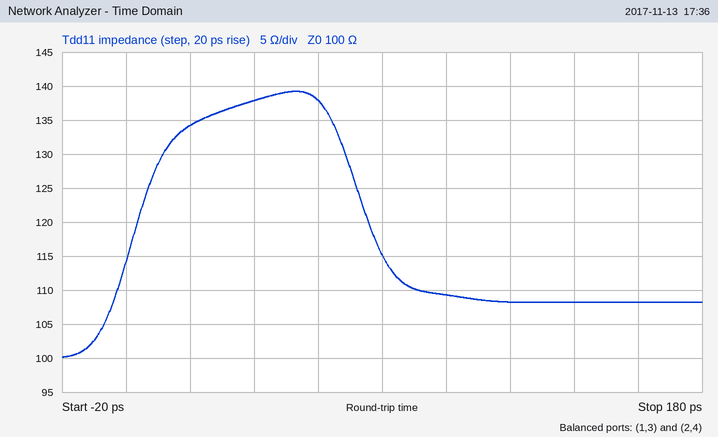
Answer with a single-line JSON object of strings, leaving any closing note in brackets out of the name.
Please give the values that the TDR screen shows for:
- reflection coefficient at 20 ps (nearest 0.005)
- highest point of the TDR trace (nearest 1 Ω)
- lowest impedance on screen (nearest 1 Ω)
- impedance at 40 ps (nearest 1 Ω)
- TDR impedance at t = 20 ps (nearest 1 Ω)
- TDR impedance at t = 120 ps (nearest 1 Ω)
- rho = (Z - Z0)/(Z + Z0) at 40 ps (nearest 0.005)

{"reflection coefficient at 20 ps": "+0.145", "highest point of the TDR trace": "139 Ω", "lowest impedance on screen": "100 Ω", "impedance at 40 ps": "138 Ω", "TDR impedance at t = 20 ps": "134 Ω", "TDR impedance at t = 120 ps": "108 Ω", "rho = (Z - Z0)/(Z + Z0) at 40 ps": "+0.160"}
